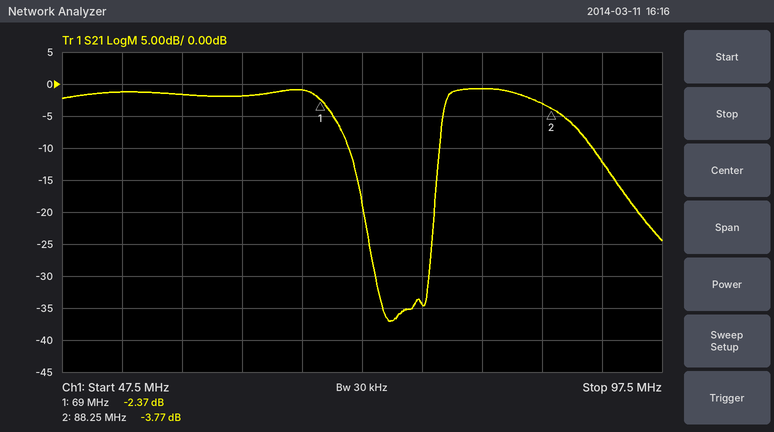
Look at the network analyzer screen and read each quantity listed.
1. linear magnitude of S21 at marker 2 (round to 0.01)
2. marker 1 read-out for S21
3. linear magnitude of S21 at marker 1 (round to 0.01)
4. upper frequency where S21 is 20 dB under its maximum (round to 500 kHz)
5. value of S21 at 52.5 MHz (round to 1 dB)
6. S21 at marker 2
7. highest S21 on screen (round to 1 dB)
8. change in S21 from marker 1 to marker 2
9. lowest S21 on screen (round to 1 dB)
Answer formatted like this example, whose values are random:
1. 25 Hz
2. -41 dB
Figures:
1. 0.65
2. -2.37 dB
3. 0.76
4. 96.0 MHz
5. -1 dB
6. -3.77 dB
7. -1 dB
8. -1.40 dB
9. -37 dB
